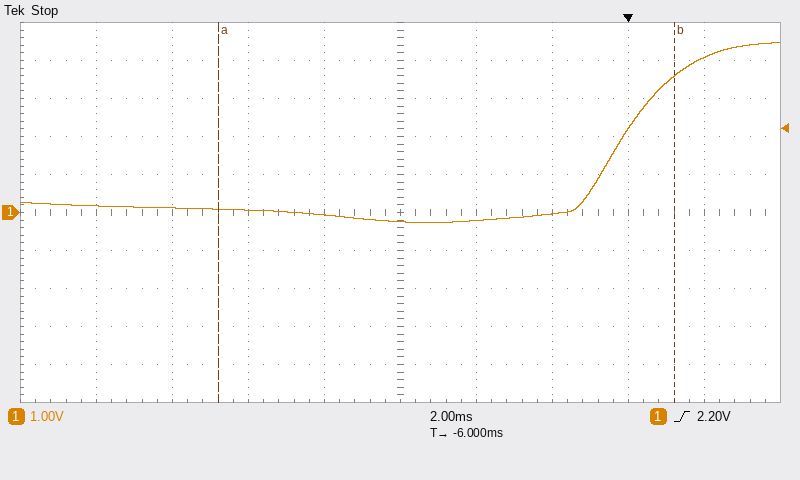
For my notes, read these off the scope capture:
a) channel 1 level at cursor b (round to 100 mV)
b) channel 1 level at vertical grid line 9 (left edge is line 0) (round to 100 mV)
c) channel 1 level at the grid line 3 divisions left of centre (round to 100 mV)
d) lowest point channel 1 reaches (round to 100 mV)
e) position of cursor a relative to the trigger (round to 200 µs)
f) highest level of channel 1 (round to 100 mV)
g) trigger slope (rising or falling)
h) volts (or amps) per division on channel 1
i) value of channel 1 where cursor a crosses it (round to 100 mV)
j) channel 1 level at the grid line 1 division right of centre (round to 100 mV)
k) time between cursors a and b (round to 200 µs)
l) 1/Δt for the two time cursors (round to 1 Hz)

3.6 V
4.1 V
100 mV
-300 mV
-10.8 ms
4.5 V
rising
1 V
100 mV
-200 mV
12.0 ms
83 Hz
